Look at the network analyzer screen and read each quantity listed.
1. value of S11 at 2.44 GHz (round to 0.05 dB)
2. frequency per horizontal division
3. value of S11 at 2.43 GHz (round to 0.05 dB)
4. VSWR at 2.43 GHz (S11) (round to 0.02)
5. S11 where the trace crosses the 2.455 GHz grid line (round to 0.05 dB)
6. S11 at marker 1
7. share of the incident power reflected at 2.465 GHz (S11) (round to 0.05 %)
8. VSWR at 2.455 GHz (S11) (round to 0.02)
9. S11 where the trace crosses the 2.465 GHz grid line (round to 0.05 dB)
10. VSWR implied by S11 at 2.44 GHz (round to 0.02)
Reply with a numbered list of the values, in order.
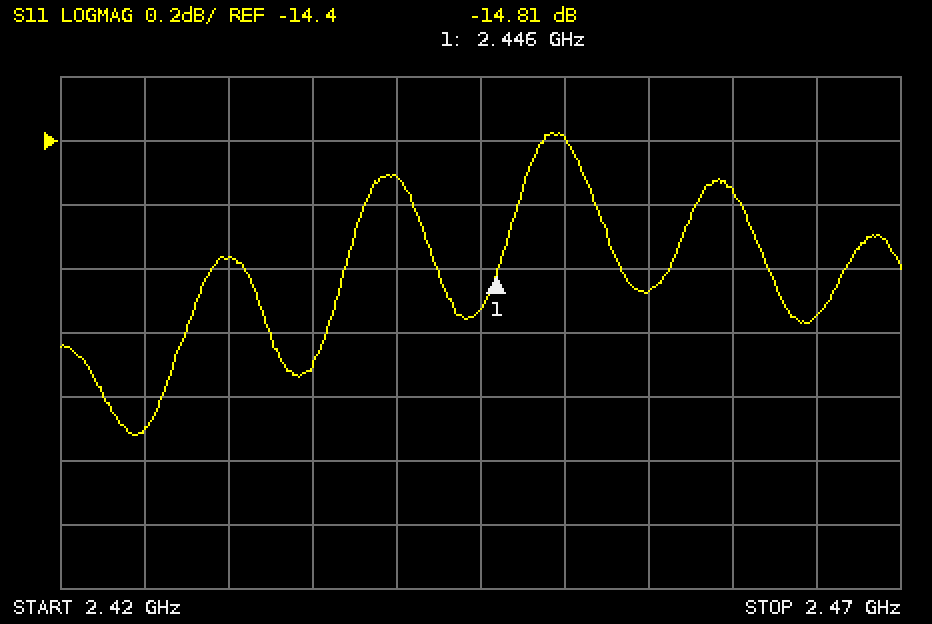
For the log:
1. -14.50 dB
2. 5 MHz
3. -14.75 dB
4. 1.44
5. -14.85 dB
6. -14.81 dB
7. 3.20 %
8. 1.44
9. -14.95 dB
10. 1.46
